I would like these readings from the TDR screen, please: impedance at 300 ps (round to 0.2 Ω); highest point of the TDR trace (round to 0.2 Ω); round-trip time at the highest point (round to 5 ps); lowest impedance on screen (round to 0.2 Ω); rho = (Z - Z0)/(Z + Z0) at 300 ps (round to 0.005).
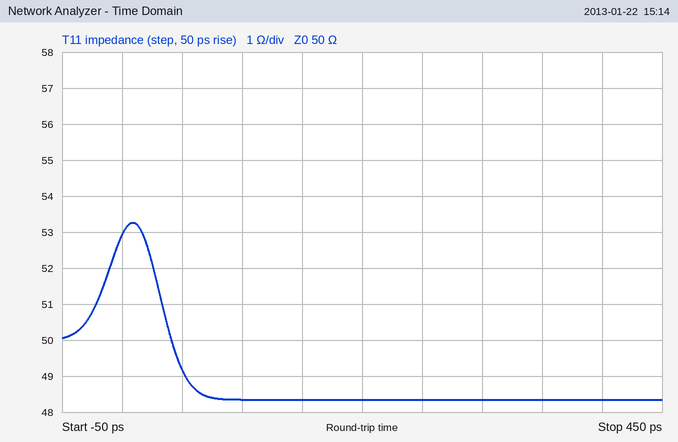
48.4 Ω
53.2 Ω
10 ps
48.4 Ω
-0.015
